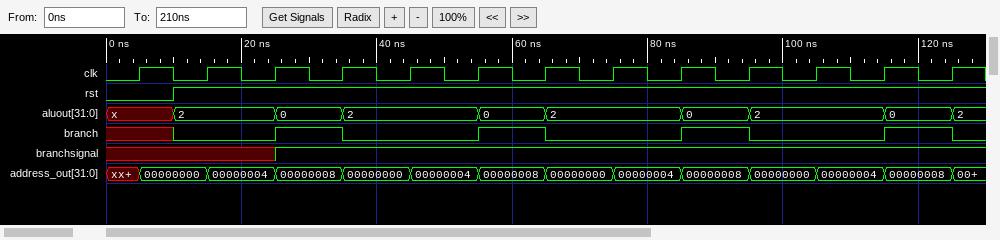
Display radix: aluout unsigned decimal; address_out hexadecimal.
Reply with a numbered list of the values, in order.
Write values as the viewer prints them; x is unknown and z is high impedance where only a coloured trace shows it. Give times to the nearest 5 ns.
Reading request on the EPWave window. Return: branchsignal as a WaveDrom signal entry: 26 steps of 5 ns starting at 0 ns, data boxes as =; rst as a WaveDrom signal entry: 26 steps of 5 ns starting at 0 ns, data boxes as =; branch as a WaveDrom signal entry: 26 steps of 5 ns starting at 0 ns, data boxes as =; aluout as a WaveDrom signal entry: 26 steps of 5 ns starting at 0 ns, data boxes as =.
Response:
1. {name: 'branchsignal', wave: 'x....1....................'}
2. {name: 'rst', wave: '0.1.......................'}
3. {name: 'branch', wave: 'x.0..1.0...1.0...1.0...1.0'}
4. {name: 'aluout', wave: 'x.=..=.=...=.=...=.=...=.=', data: '2 0 2 0 2 0 2 0 2'}
